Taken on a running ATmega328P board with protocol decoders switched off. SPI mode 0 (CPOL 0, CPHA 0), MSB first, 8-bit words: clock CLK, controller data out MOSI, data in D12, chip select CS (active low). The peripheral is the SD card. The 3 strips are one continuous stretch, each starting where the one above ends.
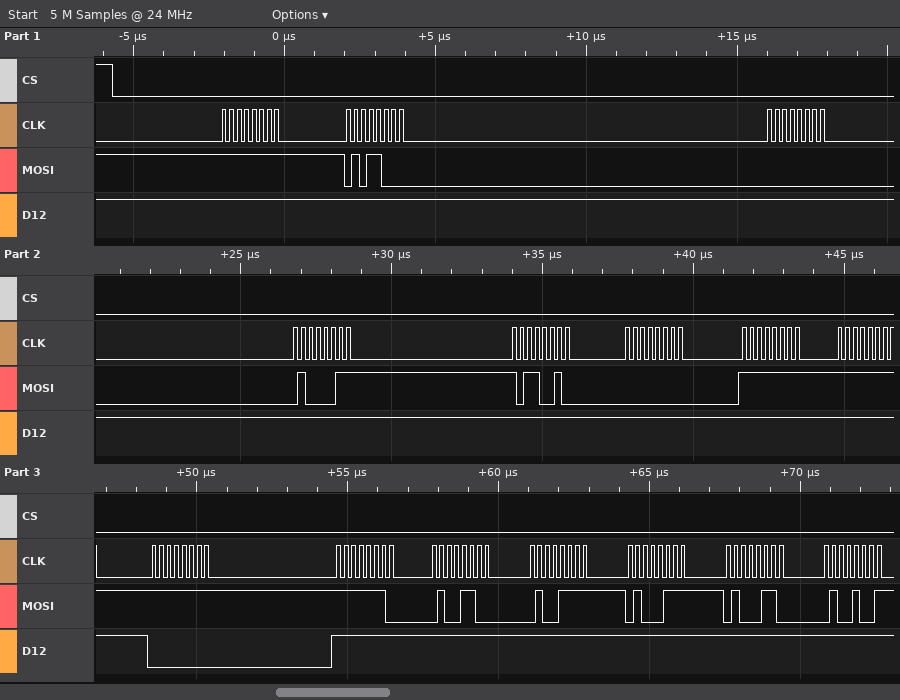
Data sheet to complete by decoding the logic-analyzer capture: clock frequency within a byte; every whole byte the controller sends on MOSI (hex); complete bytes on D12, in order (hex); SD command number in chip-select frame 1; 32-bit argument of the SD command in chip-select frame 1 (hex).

4 MHz
FF 58 00 43 B2 00 FF FF FF FE 4C 4F 47 46 49
FF FF FF FF FF FF FF FF 00 FF FF FF FF FF FF
CMD24
0x0043B200
